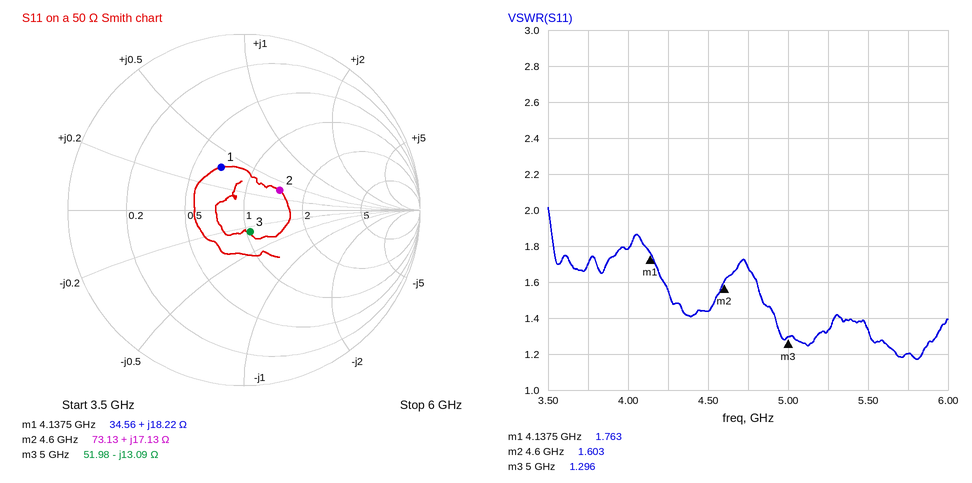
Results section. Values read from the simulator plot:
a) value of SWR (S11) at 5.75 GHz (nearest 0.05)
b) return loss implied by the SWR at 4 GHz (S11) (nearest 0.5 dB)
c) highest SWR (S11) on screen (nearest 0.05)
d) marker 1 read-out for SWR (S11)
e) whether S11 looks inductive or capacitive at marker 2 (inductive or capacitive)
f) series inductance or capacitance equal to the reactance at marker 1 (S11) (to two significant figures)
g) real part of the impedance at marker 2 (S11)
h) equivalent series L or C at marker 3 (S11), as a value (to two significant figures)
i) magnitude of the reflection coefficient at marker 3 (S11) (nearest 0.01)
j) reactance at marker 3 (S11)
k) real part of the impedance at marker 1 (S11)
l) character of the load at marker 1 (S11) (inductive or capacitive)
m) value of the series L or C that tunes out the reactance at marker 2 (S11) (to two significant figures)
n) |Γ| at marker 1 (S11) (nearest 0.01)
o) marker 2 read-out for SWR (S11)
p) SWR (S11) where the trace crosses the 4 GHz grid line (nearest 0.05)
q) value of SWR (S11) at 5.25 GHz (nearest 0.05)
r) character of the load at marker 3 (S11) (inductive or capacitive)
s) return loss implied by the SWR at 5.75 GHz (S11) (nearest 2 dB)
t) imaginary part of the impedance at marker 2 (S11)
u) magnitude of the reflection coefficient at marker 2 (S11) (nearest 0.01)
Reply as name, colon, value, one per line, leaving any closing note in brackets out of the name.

value of SWR (S11) at 5.75 GHz: 1.20
return loss implied by the SWR at 4 GHz (S11): 11.0 dB
highest SWR (S11) on screen: 2.00
marker 1 read-out for SWR: 1.763
whether S11 looks inductive or capacitive at marker 2: inductive
series inductance or capacitance equal to the reactance at marker 1 (S11): 700 pH
real part of the impedance at marker 2: 73.13 Ω
equivalent series L or C at marker 3 (S11), as a value: 2.4 pF
magnitude of the reflection coefficient at marker 3 (S11): 0.13
reactance at marker 3: -13.09 Ω
real part of the impedance at marker 1: 34.56 Ω
character of the load at marker 1 (S11): inductive
value of the series L or C that tunes out the reactance at marker 2 (S11): 2.0 pF
|Γ| at marker 1 (S11): 0.28
marker 2 read-out for SWR: 1.603
SWR (S11) where the trace crosses the 4 GHz grid line: 1.80
value of SWR (S11) at 5.25 GHz: 1.35
character of the load at marker 3 (S11): capacitive
return loss implied by the SWR at 5.75 GHz (S11): 20 dB
imaginary part of the impedance at marker 2: +17.13 Ω
magnitude of the reflection coefficient at marker 2 (S11): 0.23
